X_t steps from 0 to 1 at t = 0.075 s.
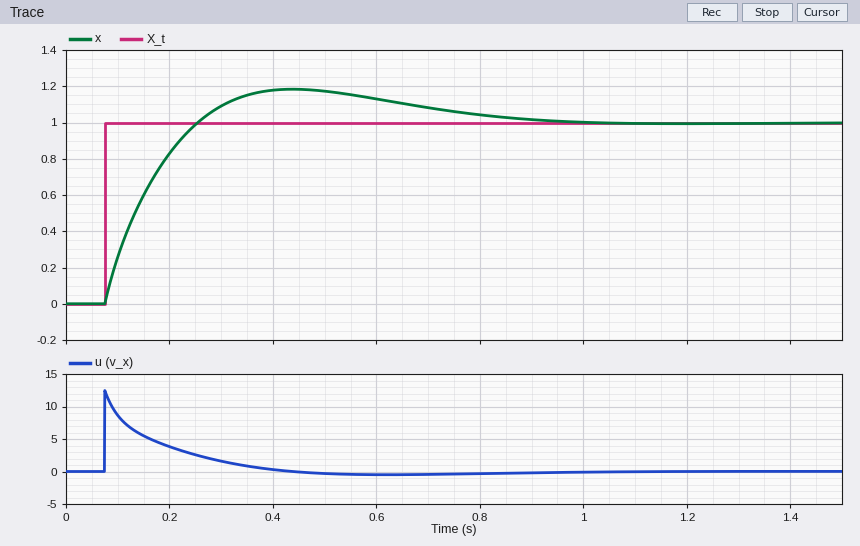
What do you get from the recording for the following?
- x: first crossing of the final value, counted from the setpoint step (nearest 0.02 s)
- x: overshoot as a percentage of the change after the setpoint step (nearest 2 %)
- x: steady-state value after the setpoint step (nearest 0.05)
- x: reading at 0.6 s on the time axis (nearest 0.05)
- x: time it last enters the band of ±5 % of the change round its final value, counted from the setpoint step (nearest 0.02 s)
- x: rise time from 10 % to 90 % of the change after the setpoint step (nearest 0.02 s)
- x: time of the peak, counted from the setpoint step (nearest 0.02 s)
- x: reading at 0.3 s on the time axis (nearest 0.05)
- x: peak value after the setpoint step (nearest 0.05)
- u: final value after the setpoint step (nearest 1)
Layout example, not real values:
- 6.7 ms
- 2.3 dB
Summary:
- 0.18 s
- 18 %
- 1.00
- 1.15
- 0.70 s
- 0.14 s
- 0.36 s
- 1.10
- 1.20
- 0
